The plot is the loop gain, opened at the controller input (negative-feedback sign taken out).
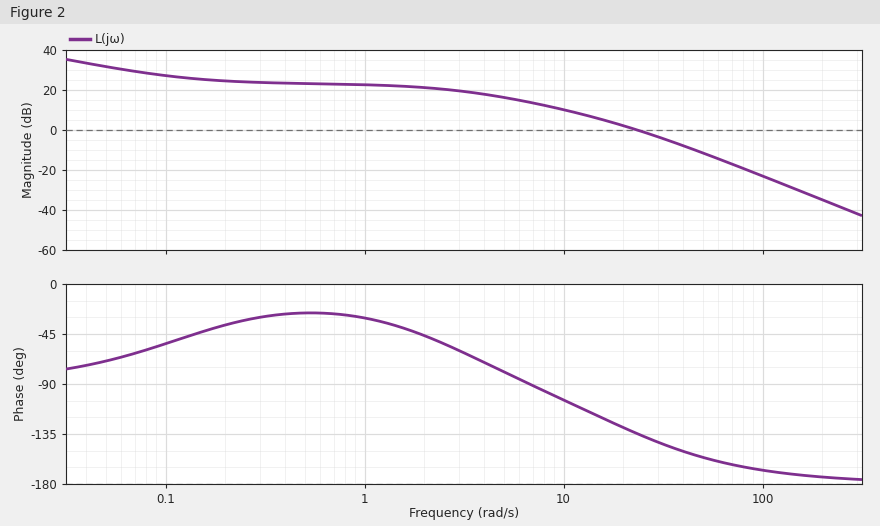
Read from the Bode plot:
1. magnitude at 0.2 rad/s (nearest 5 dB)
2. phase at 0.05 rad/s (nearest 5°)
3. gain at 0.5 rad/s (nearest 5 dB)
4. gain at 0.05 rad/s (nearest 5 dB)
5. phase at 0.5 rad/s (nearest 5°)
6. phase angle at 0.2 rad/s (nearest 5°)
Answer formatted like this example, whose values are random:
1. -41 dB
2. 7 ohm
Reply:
1. 25 dB
2. -70°
3. 25 dB
4. 30 dB
5. -25°
6. -35°
